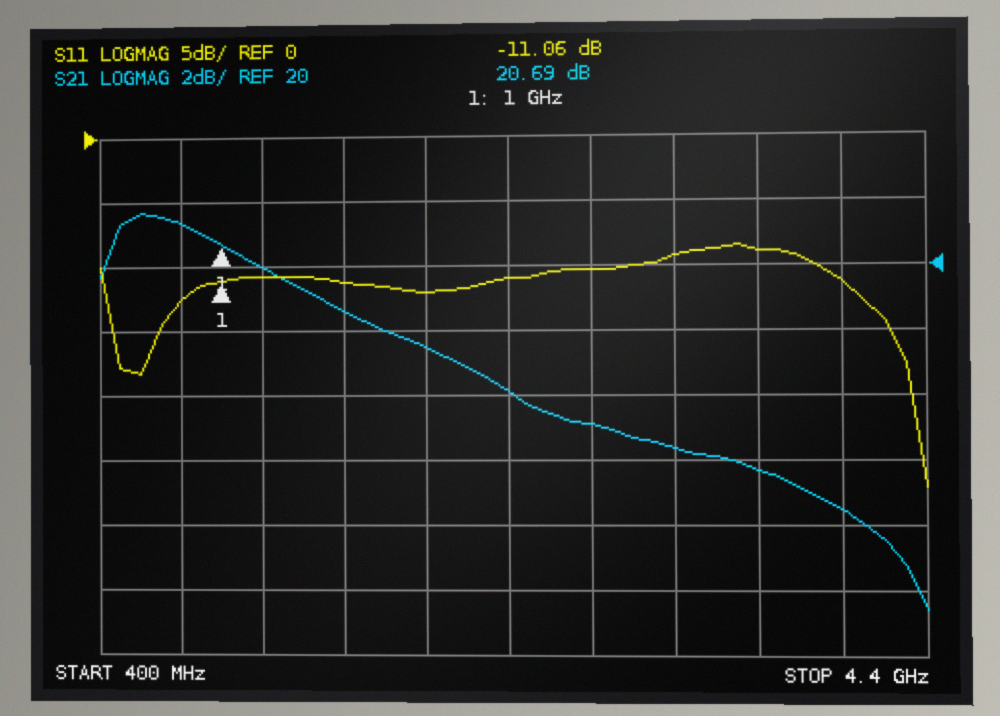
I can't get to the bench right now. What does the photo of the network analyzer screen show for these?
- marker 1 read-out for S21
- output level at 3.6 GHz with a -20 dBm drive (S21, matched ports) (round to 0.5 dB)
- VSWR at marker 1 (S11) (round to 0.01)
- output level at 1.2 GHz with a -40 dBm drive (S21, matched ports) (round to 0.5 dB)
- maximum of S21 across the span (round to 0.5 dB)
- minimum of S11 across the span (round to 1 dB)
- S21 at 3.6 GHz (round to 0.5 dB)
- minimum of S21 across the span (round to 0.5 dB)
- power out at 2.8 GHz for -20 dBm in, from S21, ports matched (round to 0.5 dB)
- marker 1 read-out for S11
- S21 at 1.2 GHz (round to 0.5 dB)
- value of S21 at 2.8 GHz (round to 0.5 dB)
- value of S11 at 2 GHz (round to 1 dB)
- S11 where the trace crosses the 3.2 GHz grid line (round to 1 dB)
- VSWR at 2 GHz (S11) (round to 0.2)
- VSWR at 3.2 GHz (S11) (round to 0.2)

20.69 dB
-6.5 dBm
1.78
-20.0 dBm
21.5 dB
-27 dB
13.5 dB
9.5 dB
-5.0 dBm
-11.06 dB
20.0 dB
15.0 dB
-12 dB
-9 dB
1.6
2.0
